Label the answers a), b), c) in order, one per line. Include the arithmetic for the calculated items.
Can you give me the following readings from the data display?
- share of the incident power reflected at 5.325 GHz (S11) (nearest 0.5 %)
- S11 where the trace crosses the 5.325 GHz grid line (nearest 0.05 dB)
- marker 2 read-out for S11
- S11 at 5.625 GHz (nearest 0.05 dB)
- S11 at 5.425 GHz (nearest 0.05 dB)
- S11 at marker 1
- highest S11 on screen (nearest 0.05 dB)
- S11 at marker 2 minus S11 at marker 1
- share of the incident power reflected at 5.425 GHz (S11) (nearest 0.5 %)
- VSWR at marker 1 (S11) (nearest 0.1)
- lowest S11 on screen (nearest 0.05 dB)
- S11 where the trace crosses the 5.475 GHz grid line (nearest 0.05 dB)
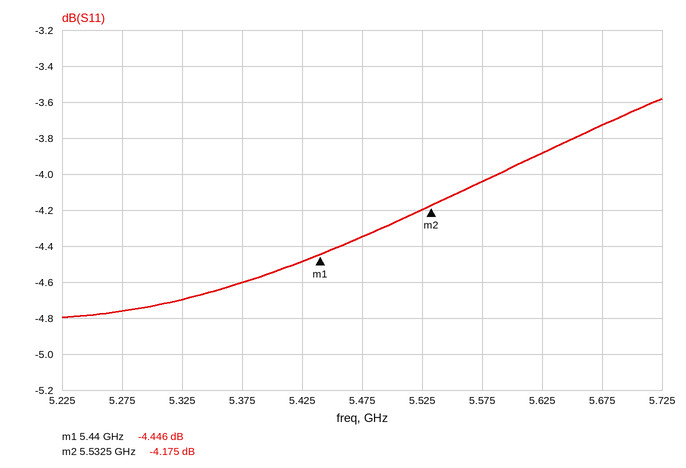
a) 10^(-4.7/10) ≈ 33.9 %, so 34.0 % to the nearest 0.5 %
b) -4.70 dB
c) -4.175 dB
d) -3.90 dB
e) -4.50 dB
f) -4.446 dB
g) -3.60 dB
h) -4.175 − (-4.446) = 0.271 dB
i) 10^(-4.5/10) ≈ 35.5 %
j) (1 + 0.5994)/(1 − 0.5994) ≈ 4.0
k) -4.80 dB
l) -4.35 dB
